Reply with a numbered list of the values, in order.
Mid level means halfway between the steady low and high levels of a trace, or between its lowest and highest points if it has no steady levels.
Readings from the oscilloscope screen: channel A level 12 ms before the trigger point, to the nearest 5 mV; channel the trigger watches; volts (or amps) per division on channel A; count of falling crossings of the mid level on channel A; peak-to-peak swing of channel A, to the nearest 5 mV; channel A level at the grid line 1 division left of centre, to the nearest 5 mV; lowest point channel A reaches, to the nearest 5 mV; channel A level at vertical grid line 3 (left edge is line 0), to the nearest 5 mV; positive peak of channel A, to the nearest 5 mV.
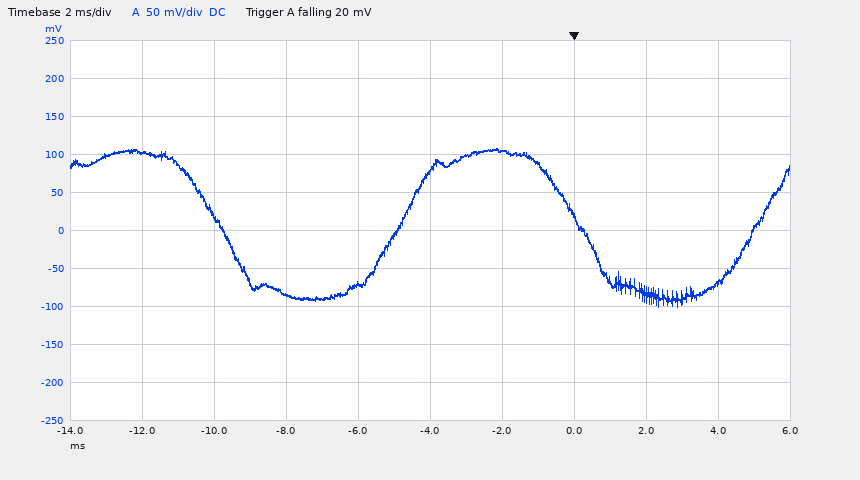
1. 100 mV
2. channel A
3. 50 mV
4. 2
5. 210 mV
6. -70 mV
7. -100 mV
8. -85 mV
9. 110 mV
